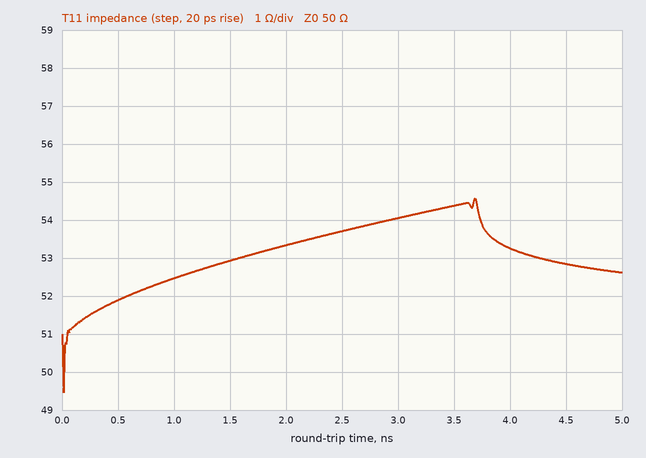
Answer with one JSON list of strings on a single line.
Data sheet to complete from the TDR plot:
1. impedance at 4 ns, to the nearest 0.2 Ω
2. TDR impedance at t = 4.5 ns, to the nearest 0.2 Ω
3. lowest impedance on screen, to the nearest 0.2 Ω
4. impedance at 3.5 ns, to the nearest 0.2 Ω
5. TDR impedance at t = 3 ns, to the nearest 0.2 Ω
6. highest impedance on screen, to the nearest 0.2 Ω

["53.2 Ω", "52.8 Ω", "49.4 Ω", "54.4 Ω", "54.0 Ω", "54.6 Ω"]
